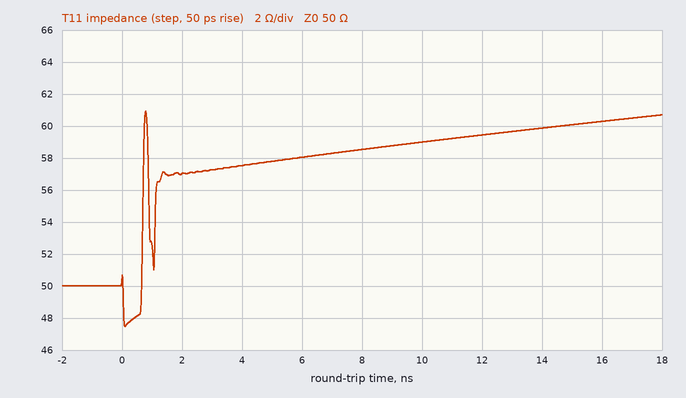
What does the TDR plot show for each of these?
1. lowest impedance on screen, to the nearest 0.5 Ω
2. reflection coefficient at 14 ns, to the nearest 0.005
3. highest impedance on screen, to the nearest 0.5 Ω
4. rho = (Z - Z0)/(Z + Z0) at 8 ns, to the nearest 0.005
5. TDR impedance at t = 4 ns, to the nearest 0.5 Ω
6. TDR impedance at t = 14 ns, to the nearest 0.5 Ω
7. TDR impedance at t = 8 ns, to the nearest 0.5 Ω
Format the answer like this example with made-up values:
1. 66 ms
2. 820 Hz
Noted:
1. 47.5 Ω
2. +0.090
3. 61.0 Ω
4. +0.080
5. 57.5 Ω
6. 60.0 Ω
7. 58.5 Ω
